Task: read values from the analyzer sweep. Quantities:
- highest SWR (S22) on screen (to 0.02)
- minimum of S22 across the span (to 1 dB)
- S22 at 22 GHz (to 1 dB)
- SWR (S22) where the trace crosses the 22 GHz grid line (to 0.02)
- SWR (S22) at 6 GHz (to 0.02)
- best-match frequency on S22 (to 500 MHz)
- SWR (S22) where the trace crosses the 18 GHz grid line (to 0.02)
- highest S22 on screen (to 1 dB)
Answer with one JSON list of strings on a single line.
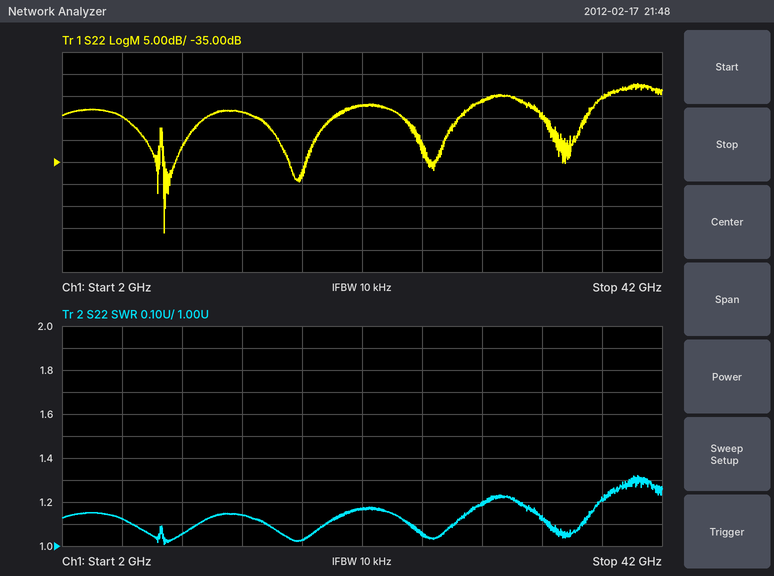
["1.32", "-51 dB", "-22 dB", "1.16", "1.12", "9.0 GHz", "1.02", "-17 dB"]
